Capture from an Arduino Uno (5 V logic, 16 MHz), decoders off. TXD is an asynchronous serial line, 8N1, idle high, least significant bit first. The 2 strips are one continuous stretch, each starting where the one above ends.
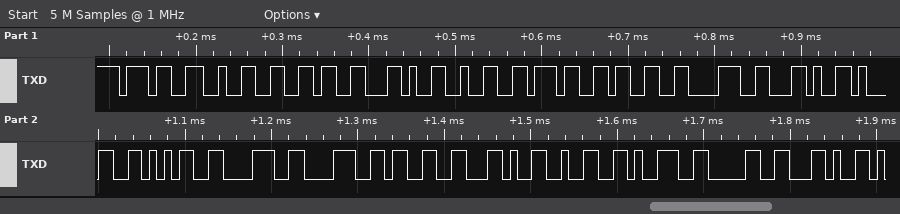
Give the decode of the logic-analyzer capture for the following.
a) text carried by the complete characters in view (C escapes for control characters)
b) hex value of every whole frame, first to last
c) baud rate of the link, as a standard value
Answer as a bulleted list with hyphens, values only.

- "726,2738,15883,290,"
- 0x37 0x32 0x36 0x2C 0x32 0x37 0x33 0x38 0x2C 0x31 0x35 0x38 0x38 0x33 0x2C 0x32 0x39 0x30 0x2C
- 115200 baud
